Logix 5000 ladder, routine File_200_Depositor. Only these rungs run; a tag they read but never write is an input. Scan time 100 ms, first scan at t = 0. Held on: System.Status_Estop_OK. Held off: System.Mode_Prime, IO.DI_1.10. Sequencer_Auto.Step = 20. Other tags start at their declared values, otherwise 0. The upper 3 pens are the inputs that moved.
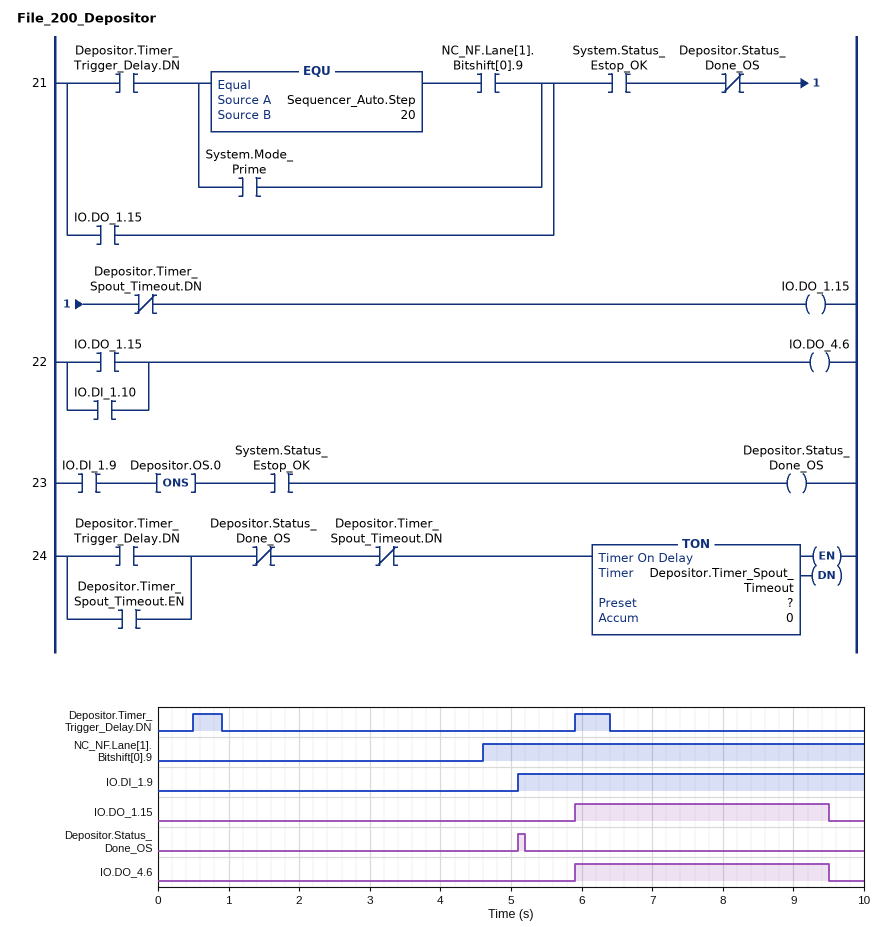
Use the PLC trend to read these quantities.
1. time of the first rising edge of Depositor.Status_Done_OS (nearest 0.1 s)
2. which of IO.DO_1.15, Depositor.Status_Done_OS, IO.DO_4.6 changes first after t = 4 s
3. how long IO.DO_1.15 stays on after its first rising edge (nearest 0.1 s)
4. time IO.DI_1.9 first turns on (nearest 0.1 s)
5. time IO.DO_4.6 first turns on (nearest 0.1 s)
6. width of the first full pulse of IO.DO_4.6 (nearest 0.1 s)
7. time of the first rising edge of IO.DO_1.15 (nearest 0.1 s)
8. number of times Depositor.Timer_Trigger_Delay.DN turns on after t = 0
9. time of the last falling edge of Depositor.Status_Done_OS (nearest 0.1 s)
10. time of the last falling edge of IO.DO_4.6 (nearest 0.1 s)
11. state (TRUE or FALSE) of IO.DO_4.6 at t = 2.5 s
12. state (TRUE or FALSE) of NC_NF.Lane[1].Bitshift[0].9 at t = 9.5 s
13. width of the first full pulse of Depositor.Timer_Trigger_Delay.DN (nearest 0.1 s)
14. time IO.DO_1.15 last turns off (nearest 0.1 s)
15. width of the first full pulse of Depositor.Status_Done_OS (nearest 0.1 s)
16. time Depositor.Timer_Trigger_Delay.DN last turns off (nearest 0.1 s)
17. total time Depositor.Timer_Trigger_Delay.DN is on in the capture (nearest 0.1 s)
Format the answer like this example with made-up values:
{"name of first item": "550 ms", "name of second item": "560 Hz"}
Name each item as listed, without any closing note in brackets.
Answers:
{"time of the first rising edge of Depositor.Status_Done_OS": "5.1 s", "which of IO.DO_1.15, Depositor.Status_Done_OS, IO.DO_4.6 changes first after t = 4 s": "Depositor.Status_Done_OS", "how long IO.DO_1.15 stays on after its first rising edge": "3.6 s", "time IO.DI_1.9 first turns on": "5.1 s", "time IO.DO_4.6 first turns on": "5.9 s", "width of the first full pulse of IO.DO_4.6": "3.6 s", "time of the first rising edge of IO.DO_1.15": "5.9 s", "number of times Depositor.Timer_Trigger_Delay.DN turns on after t = 0": "2", "time of the last falling edge of Depositor.Status_Done_OS": "5.2 s", "time of the last falling edge of IO.DO_4.6": "9.5 s", "state (TRUE or FALSE) of IO.DO_4.6 at t = 2.5 s": "FALSE", "state (TRUE or FALSE) of NC_NF.Lane[1].Bitshift[0].9 at t = 9.5 s": "TRUE", "width of the first full pulse of Depositor.Timer_Trigger_Delay.DN": "0.4 s", "time IO.DO_1.15 last turns off": "9.5 s", "width of the first full pulse of Depositor.Status_Done_OS": "0.1 s", "time Depositor.Timer_Trigger_Delay.DN last turns off": "6.4 s", "total time Depositor.Timer_Trigger_Delay.DN is on in the capture": "0.9 s"}
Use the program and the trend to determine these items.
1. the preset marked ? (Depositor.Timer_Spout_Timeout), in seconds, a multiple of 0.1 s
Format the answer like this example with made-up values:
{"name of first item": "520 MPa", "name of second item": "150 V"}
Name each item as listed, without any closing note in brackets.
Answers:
{"the preset marked ? (Depositor.Timer_Spout_Timeout), in seconds, a multiple of 0.1 s": "3.5 s"}
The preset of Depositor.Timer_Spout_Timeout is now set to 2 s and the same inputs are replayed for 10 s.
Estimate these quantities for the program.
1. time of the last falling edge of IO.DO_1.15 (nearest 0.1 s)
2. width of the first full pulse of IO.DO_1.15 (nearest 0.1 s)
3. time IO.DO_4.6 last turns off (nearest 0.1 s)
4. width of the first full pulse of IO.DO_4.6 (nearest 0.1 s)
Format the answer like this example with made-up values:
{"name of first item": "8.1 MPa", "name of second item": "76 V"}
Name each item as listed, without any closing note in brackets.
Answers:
{"time of the last falling edge of IO.DO_1.15": "8.0 s", "width of the first full pulse of IO.DO_1.15": "2.1 s", "time IO.DO_4.6 last turns off": "8.0 s", "width of the first full pulse of IO.DO_4.6": "2.1 s"}
